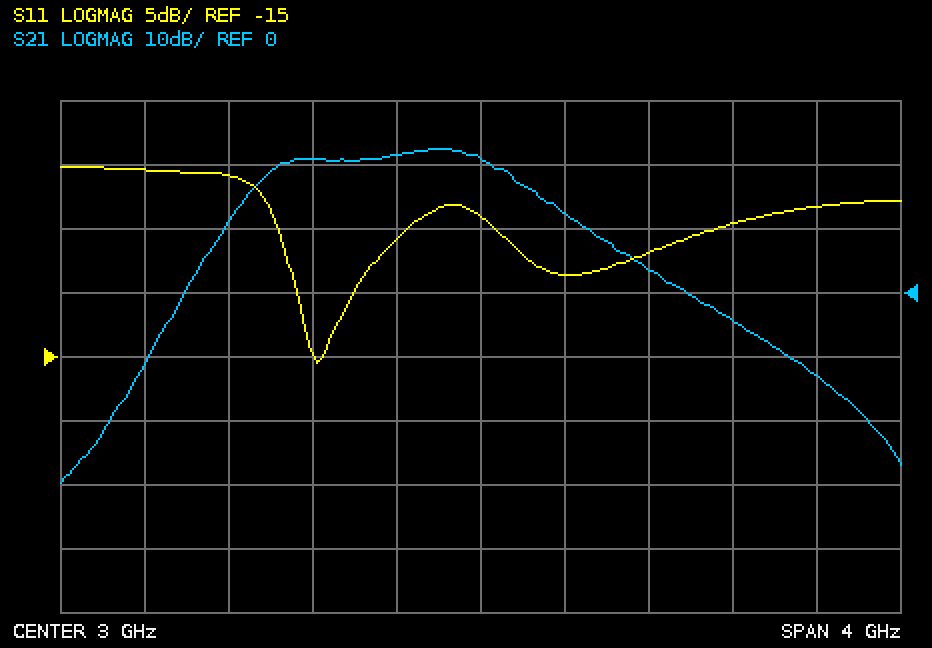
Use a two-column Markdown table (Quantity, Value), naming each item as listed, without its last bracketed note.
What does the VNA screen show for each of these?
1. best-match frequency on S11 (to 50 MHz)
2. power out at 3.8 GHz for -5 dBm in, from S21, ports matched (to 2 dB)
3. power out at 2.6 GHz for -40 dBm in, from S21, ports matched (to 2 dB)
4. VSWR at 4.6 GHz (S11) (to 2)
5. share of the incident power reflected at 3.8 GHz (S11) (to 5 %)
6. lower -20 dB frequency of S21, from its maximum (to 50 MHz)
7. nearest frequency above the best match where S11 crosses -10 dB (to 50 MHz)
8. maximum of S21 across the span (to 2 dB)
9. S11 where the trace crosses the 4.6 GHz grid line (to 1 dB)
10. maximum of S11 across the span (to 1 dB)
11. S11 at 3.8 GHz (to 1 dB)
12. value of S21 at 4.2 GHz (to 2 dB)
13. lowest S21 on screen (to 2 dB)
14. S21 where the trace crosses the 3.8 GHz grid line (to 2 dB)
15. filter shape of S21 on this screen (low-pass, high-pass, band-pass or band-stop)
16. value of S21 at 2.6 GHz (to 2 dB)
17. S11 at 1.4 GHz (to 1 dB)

| Quantity | Value |
|---|---|
| best-match frequency on S11 | 2.20 GHz |
| power out at 3.8 GHz for -5 dBm in, from S21, ports matched | -2 dBm |
| power out at 2.6 GHz for -40 dBm in, from S21, ports matched | -18 dBm |
| VSWR at 4.6 GHz (S11) | 6 |
| share of the incident power reflected at 3.8 GHz (S11) | 20 % |
| lower -20 dB frequency of S21, from its maximum | 1.65 GHz |
| nearest frequency above the best match where S11 crosses -10 dB | 2.40 GHz |
| maximum of S21 across the span | 22 dB |
| S11 where the trace crosses the 4.6 GHz grid line | -3 dB |
| maximum of S11 across the span | 0 dB |
| S11 at 3.8 GHz | -7 dB |
| value of S21 at 4.2 GHz | -4 dB |
| lowest S21 on screen | -30 dB |
| S21 where the trace crosses the 3.8 GHz grid line | 4 dB |
| filter shape of S21 on this screen | band-pass |
| value of S21 at 2.6 GHz | 22 dB |
| S11 at 1.4 GHz | 0 dB |
